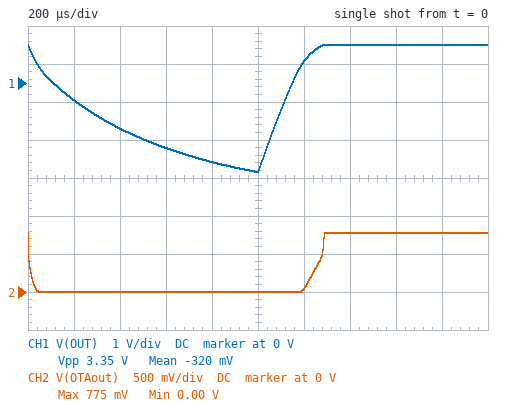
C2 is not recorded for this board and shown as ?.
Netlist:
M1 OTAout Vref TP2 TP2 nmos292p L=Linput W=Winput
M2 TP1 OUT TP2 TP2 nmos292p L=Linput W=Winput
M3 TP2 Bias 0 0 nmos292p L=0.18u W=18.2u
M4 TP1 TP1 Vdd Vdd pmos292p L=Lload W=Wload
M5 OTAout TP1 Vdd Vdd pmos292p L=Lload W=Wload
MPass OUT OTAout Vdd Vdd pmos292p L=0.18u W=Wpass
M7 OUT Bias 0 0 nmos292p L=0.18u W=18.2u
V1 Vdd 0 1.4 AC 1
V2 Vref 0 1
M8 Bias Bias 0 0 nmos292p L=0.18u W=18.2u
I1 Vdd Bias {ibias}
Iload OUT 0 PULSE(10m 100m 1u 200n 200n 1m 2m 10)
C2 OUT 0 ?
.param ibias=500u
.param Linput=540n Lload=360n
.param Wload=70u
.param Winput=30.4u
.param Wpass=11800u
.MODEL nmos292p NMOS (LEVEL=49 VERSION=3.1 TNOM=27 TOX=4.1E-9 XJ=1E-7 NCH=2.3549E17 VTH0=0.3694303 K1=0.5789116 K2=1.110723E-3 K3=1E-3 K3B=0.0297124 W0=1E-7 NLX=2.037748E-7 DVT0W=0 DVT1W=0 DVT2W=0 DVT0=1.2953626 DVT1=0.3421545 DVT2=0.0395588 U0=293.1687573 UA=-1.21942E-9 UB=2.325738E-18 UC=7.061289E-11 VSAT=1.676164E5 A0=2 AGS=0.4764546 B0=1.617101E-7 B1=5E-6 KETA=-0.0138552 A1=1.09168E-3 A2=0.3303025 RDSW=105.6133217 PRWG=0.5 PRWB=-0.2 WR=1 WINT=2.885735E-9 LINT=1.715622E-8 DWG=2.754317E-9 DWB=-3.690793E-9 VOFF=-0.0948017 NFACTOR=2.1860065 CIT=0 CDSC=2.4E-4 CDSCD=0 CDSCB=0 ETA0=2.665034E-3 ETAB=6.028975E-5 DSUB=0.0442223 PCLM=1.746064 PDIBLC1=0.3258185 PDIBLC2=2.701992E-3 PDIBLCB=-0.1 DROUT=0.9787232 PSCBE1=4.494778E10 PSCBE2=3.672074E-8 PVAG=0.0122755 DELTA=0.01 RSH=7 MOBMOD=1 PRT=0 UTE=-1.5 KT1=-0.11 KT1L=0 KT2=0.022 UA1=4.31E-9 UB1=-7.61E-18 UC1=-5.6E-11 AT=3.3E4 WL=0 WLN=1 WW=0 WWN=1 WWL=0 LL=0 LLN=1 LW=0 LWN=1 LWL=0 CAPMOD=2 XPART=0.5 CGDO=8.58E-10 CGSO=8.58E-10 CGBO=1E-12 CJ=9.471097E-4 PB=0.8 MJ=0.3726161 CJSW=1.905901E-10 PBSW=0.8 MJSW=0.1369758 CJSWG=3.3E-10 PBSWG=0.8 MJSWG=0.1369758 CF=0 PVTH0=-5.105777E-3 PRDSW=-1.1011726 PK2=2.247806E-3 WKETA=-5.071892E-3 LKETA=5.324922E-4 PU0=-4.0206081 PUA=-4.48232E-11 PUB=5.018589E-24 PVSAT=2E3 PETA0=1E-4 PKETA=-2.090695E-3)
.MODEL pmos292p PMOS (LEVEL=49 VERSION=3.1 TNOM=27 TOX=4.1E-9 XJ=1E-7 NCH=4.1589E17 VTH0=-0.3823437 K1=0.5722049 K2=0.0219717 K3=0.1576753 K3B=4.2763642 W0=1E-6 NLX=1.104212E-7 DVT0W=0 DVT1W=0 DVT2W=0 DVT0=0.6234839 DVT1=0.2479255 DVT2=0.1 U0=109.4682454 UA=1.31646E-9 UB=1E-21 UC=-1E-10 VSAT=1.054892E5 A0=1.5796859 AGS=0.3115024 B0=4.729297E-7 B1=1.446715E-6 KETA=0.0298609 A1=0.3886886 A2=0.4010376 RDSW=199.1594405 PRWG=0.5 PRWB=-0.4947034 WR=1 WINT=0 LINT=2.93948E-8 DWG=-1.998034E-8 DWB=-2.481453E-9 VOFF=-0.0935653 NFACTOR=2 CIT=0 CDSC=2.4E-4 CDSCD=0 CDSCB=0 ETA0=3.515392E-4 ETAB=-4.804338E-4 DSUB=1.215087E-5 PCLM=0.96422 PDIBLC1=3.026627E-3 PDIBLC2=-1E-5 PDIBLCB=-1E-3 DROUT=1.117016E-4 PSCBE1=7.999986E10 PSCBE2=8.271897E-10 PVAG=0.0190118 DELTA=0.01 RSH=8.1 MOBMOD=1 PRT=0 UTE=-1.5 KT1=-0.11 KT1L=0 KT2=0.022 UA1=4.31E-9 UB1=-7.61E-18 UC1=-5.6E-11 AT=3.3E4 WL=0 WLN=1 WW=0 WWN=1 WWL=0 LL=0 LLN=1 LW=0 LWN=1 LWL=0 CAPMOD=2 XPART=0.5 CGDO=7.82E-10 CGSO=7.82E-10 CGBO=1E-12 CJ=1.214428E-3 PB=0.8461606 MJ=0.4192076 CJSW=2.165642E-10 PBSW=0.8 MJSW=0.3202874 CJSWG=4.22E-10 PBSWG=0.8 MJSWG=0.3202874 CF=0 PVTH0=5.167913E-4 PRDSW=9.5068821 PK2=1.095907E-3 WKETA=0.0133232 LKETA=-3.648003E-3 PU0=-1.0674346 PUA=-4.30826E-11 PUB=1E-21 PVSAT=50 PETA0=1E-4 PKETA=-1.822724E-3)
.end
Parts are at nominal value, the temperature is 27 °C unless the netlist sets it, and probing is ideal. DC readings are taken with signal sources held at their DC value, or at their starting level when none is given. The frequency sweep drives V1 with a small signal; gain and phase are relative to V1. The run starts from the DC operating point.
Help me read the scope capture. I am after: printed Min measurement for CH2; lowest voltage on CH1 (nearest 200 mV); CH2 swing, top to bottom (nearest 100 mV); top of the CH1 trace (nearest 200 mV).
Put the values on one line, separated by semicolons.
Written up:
0.00 V; -2.4 V; 800 mV; 1.0 V
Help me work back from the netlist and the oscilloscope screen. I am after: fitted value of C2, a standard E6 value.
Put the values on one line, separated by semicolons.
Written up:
4.7 µF
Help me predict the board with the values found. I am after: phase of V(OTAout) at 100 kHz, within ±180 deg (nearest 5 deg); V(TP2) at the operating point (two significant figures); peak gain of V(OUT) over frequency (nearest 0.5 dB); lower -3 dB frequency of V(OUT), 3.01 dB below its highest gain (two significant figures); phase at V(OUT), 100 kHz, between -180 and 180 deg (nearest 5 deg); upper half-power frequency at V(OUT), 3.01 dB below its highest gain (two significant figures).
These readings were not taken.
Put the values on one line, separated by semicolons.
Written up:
-5 deg; 370 mV; -53.0 dB; 56 kHz; 10 deg; 480 kHz
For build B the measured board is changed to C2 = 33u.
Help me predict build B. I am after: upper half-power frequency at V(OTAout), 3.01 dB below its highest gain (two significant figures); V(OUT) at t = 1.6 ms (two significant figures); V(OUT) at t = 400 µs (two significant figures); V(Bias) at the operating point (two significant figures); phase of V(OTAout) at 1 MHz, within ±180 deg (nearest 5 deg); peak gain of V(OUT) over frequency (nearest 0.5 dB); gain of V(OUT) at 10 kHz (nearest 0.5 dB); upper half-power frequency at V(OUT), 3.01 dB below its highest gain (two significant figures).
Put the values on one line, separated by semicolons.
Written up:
680 kHz; 720 mV; 340 mV; 660 mV; -10 deg; -60.0 dB; -62.0 dB; 14 kHz
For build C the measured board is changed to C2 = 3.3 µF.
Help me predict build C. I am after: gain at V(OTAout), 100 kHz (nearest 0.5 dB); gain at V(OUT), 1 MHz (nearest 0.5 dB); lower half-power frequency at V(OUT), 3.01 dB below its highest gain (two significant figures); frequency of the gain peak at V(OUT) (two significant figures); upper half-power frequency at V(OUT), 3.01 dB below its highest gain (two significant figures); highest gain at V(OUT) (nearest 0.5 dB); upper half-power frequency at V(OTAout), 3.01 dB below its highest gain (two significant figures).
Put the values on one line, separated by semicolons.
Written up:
0.5 dB; -58.0 dB; 87 kHz; 220 kHz; 510 kHz; -50.0 dB; 590 kHz
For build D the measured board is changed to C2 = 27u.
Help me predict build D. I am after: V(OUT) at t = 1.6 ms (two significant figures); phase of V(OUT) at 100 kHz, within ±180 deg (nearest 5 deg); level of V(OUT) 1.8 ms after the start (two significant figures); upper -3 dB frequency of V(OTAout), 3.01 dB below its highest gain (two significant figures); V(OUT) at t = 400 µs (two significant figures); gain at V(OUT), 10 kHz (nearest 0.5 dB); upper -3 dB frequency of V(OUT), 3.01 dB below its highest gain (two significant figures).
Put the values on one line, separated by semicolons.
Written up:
770 mV; -25 deg; 930 mV; 680 kHz; 240 mV; -61.0 dB; 18 kHz
